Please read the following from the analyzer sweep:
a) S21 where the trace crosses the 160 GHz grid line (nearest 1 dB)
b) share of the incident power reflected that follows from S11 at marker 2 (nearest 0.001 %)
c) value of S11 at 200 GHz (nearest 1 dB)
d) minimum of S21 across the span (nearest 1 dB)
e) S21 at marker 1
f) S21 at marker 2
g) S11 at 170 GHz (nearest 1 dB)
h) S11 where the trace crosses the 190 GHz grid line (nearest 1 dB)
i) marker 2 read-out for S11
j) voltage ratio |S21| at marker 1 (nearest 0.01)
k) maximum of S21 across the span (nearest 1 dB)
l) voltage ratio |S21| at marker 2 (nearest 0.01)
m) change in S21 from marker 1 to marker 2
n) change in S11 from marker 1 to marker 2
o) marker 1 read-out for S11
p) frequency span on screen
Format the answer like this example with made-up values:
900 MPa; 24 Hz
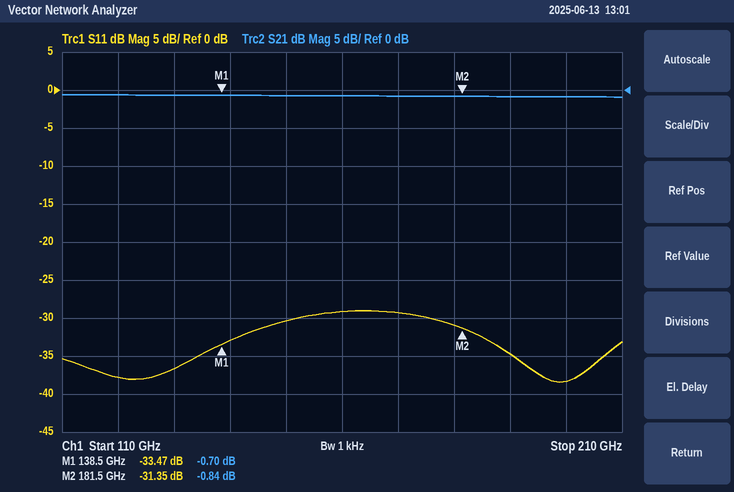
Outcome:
-1 dB; 0.073 %; -38 dB; -1 dB; -0.70 dB; -0.84 dB; -29 dB; -35 dB; -31.35 dB; 0.92; -1 dB; 0.91; -0.14 dB; 2.12 dB; -33.47 dB; 100 GHz
